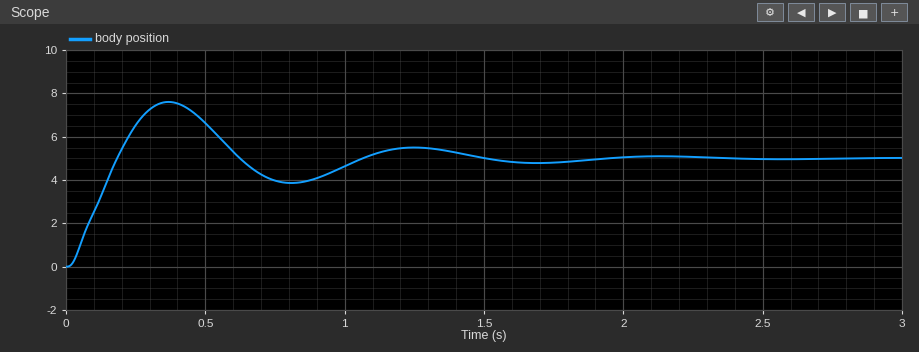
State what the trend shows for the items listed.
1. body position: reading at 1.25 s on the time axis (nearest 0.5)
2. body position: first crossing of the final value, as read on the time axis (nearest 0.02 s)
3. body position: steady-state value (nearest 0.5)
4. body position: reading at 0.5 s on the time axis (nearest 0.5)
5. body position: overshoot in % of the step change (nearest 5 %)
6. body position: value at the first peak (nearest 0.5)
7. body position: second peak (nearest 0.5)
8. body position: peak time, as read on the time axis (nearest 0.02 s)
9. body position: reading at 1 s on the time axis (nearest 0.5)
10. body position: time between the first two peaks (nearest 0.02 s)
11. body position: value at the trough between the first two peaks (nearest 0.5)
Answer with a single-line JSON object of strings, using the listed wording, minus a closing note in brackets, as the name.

{"body position: reading at 1.25 s on the time axis": "5.5", "body position: first crossing of the final value, as read on the time axis": "0.18 s", "body position: steady-state value": "5.0", "body position: reading at 0.5 s on the time axis": "6.5", "body position: overshoot in % of the step change": "50 %", "body position: value at the first peak": "7.5", "body position: second peak": "5.5", "body position: peak time, as read on the time axis": "0.36 s", "body position: reading at 1 s on the time axis": "4.5", "body position: time between the first two peaks": "0.88 s", "body position: value at the trough between the first two peaks": "4.0"}
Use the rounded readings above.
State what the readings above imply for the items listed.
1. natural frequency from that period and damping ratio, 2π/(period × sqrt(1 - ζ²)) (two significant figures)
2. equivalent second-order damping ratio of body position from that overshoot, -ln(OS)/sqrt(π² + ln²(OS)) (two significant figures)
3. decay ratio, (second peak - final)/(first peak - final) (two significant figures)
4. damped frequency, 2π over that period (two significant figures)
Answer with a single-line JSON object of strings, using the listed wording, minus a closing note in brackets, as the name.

{"natural frequency from that period and damping ratio, 2π/(period × sqrt(1 - ζ²))": "7.3 rad/s", "equivalent second-order damping ratio of body position from that overshoot, -ln(OS)/sqrt(π² + ln²(OS))": "0.22", "decay ratio, (second peak - final)/(first peak - final)": "0.20", "damped frequency, 2π over that period": "7.1 rad/s"}
